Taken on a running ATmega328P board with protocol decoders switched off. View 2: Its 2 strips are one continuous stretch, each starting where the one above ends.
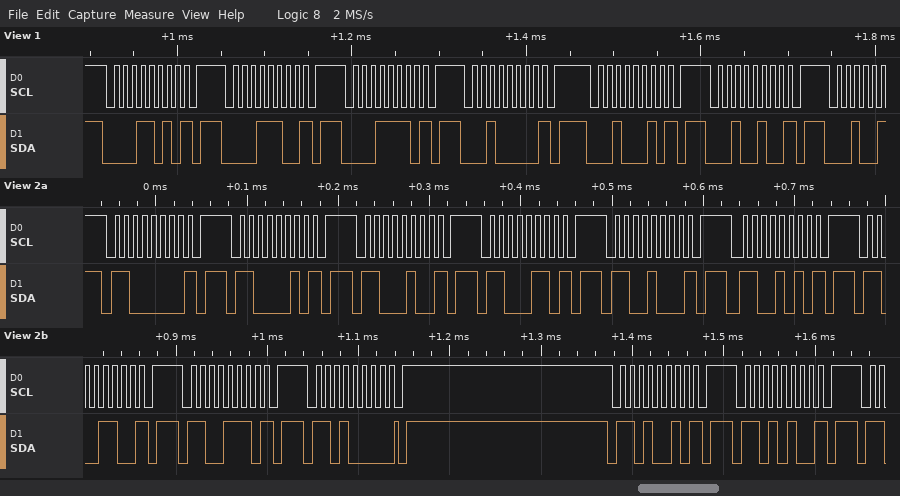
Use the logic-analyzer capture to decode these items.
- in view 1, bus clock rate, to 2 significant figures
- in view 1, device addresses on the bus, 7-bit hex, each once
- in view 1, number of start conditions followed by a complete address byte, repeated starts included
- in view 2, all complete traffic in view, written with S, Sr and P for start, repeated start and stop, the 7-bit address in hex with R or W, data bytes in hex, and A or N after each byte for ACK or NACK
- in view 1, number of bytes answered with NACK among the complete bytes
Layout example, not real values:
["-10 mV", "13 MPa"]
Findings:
["100 kHz", "0x0D 0x0E 0x0F 0x10 0x11 0x12", "6", "S 60W N P S 61W N P S 62W N P S 63W N P S 64W N P S 65W N P S 66W N P S 67W N P S 68W A P S 69W N P S 6AW N P", "6"]
